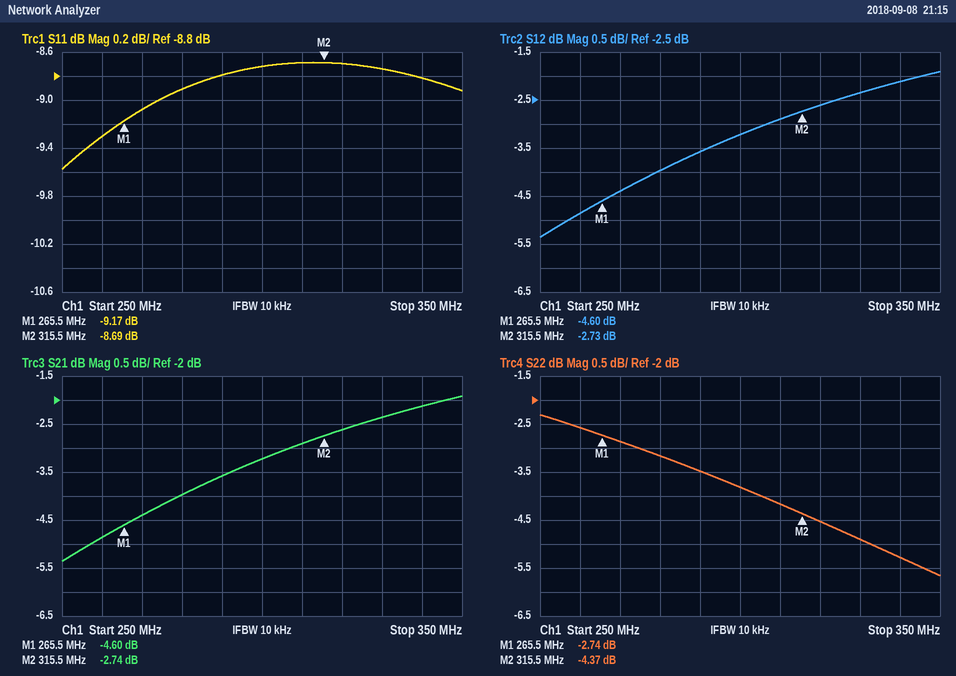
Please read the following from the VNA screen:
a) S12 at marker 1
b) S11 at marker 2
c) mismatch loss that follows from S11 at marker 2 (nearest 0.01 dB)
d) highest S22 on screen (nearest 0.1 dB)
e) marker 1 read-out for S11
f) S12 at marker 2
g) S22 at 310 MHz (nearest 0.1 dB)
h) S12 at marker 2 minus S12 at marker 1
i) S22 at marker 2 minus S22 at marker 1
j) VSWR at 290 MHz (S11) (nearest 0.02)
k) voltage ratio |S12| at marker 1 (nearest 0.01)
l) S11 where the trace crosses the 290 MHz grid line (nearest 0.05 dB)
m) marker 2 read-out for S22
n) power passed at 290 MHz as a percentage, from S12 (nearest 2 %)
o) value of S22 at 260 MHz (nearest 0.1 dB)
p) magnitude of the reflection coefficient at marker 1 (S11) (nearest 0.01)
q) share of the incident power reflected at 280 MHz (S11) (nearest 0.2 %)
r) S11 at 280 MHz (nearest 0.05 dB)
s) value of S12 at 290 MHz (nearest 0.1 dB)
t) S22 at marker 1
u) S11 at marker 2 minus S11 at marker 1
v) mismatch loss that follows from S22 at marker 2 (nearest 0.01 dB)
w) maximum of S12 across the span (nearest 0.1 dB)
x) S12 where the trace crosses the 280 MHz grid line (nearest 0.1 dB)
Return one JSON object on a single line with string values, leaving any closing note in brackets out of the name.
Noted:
{"S12 at marker 1": "-4.60 dB", "S11 at marker 2": "-8.69 dB", "mismatch loss that follows from S11 at marker 2": "0.63 dB", "highest S22 on screen": "-2.3 dB", "marker 1 read-out for S11": "-9.17 dB", "S12 at marker 2": "-2.73 dB", "S22 at 310 MHz": "-4.2 dB", "S12 at marker 2 minus S12 at marker 1": "1.87 dB", "S22 at marker 2 minus S22 at marker 1": "-1.63 dB", "VSWR at 290 MHz (S11)": "2.14", "voltage ratio |S12| at marker 1": "0.59", "S11 where the trace crosses the 290 MHz grid line": "-8.80 dB", "marker 2 read-out for S22": "-4.37 dB", "power passed at 290 MHz as a percentage, from S12": "44 %", "value of S22 at 260 MHz": "-2.6 dB", "magnitude of the reflection coefficient at marker 1 (S11)": "0.35", "share of the incident power reflected at 280 MHz (S11)": "12.8 %", "S11 at 280 MHz": "-8.90 dB", "value of S12 at 290 MHz": "-3.6 dB", "S22 at marker 1": "-2.74 dB", "S11 at marker 2 minus S11 at marker 1": "0.48 dB", "mismatch loss that follows from S22 at marker 2": "1.98 dB", "maximum of S12 across the span": "-1.9 dB", "S12 where the trace crosses the 280 MHz grid line": "-4.0 dB"}
